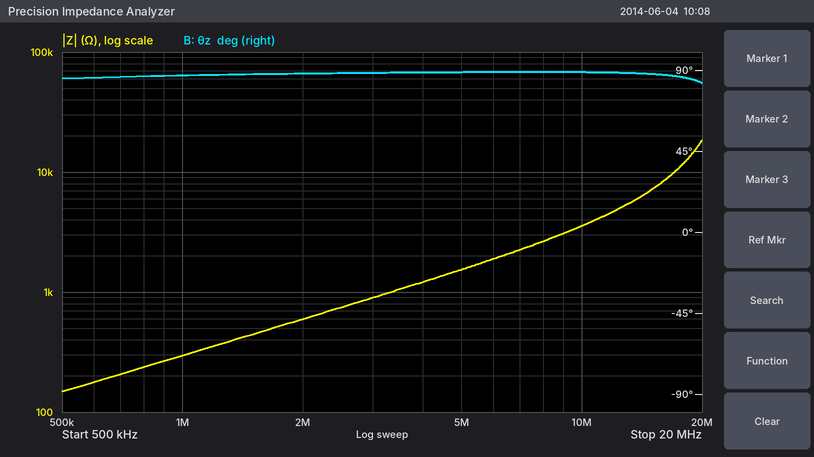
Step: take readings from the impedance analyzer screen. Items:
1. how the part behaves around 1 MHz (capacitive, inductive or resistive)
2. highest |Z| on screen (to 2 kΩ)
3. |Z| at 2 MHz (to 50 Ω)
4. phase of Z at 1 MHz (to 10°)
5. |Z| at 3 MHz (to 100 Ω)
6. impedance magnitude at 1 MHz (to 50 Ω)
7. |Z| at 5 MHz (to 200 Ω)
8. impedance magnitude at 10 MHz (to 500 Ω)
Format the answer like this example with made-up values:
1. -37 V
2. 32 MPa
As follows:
1. inductive
2. 18 kΩ
3. 600 Ω
4. 90°
5. 900 Ω
6. 300 Ω
7. 1.6 kΩ
8. 3.5 kΩ
